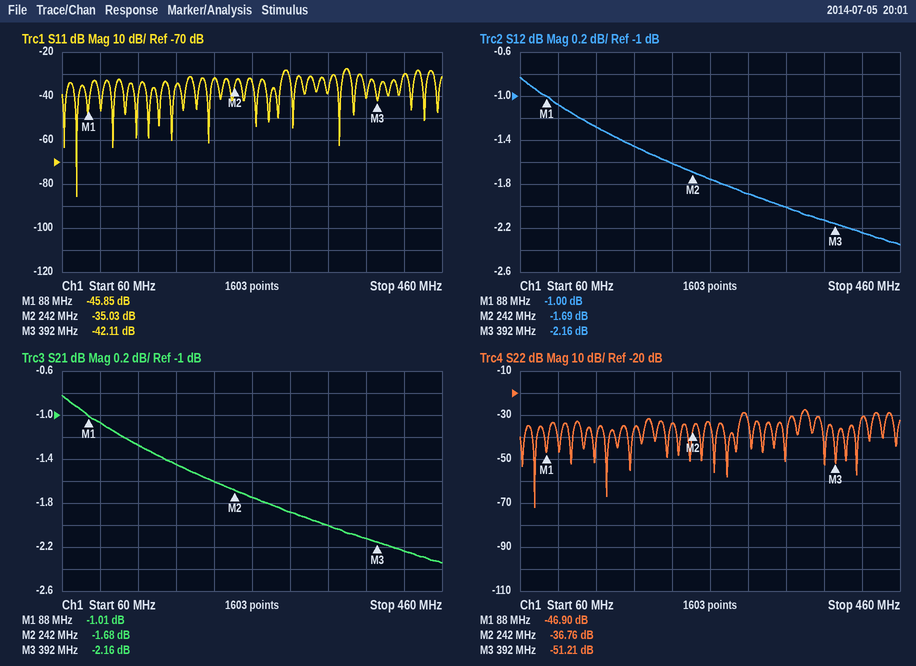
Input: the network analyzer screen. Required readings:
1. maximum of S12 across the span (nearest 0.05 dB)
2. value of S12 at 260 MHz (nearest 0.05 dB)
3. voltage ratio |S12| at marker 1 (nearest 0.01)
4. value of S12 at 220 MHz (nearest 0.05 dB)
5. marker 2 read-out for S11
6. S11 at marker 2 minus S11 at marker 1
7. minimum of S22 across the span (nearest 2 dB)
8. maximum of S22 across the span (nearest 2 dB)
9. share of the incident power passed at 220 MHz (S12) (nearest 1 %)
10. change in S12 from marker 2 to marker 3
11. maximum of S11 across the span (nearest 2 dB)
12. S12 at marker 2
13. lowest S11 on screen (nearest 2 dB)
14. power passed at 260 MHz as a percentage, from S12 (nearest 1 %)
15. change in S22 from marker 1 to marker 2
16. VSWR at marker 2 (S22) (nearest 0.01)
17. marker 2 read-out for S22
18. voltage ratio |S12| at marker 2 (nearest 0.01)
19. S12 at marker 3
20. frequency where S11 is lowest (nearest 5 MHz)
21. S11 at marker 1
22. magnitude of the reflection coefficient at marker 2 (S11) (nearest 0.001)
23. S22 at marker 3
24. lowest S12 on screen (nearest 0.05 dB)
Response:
-0.85 dB
-1.75 dB
0.89
-1.60 dB
-35.03 dB
10.82 dB
-72 dB
-28 dB
69 %
-0.47 dB
-28 dB
-1.69 dB
-86 dB
67 %
10.14 dB
1.03
-36.76 dB
0.82
-2.16 dB
75 MHz
-45.85 dB
0.018
-51.21 dB
-2.35 dB
